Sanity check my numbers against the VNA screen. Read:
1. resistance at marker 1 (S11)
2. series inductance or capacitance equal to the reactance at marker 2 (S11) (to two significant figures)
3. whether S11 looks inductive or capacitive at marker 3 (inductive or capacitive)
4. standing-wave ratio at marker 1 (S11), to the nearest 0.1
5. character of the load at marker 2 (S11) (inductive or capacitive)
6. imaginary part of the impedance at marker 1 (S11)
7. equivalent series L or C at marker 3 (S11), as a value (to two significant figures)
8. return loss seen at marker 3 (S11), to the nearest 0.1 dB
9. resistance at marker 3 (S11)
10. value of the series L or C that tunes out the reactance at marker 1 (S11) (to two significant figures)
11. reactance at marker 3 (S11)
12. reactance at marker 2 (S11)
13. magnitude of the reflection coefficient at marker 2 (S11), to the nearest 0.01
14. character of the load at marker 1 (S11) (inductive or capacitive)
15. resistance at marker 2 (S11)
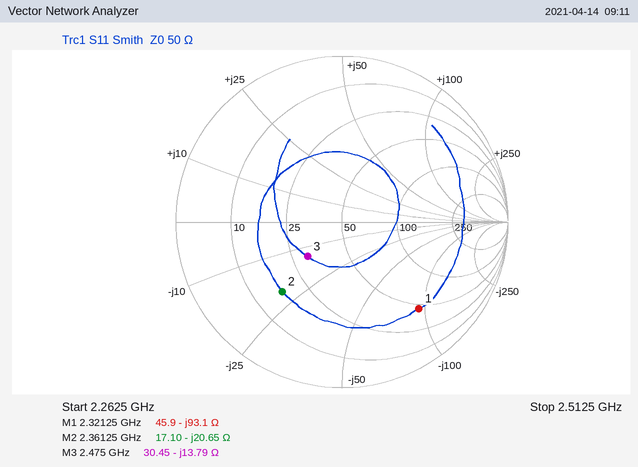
45.9 Ω
3.3 pF
capacitive
5.6
capacitive
-93.1 Ω
4.7 pF
10.7 dB
30.45 Ω
6.4 nH
-13.79 Ω
-20.65 Ω
0.55
capacitive
17.10 Ω
